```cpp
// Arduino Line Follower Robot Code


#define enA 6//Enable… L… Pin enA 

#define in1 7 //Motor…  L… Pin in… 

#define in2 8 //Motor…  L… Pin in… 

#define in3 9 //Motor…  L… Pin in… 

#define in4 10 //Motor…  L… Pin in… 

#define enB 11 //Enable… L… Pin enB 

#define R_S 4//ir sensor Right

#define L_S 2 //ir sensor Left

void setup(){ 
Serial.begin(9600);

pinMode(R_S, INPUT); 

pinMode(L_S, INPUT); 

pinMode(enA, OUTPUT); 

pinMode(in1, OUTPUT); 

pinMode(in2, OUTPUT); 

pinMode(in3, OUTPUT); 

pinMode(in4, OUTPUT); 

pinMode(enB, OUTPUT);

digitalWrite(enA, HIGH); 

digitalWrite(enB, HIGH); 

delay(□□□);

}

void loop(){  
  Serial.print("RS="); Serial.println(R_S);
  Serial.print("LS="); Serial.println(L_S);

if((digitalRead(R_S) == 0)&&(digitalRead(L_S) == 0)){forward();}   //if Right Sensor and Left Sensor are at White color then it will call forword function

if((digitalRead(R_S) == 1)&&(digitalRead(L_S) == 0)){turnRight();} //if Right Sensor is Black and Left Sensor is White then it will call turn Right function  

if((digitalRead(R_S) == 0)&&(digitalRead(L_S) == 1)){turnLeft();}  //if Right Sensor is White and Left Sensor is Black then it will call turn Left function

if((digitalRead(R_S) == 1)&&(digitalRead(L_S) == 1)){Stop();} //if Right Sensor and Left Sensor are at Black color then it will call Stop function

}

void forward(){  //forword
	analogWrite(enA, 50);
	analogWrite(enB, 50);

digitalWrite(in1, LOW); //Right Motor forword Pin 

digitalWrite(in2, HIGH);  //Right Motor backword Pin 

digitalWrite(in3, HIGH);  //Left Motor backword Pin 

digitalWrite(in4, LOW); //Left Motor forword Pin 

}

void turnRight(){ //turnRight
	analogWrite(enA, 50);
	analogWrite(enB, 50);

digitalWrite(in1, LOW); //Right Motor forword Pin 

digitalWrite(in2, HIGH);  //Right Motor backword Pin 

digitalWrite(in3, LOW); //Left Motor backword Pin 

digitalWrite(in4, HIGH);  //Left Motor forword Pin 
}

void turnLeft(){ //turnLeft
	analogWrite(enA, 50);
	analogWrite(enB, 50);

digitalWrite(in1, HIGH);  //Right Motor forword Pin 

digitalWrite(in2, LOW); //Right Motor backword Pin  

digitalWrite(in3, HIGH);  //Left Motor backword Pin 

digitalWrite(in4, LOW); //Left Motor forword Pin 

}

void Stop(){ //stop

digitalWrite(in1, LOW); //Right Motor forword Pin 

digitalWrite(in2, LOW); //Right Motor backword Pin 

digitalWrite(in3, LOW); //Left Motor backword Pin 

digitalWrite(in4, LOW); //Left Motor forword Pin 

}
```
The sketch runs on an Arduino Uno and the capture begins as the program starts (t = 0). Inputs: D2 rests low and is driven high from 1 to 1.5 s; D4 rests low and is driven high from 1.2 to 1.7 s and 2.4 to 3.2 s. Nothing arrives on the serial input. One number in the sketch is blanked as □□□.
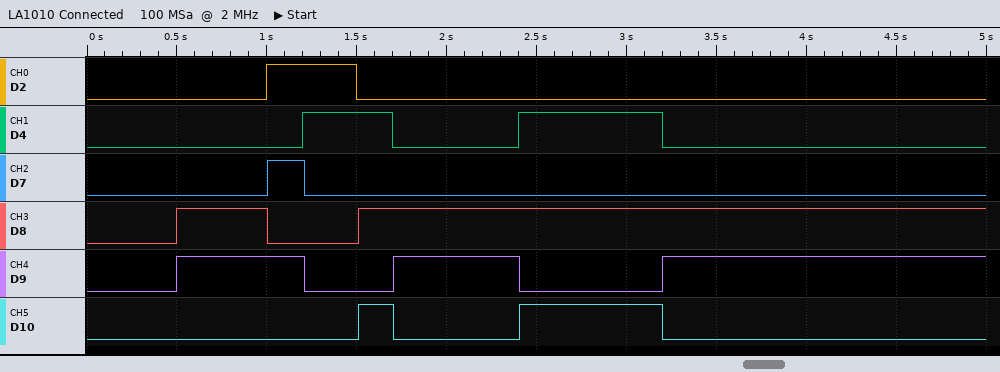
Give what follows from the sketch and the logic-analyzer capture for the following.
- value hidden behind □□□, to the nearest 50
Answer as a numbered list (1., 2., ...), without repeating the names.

1. 500
